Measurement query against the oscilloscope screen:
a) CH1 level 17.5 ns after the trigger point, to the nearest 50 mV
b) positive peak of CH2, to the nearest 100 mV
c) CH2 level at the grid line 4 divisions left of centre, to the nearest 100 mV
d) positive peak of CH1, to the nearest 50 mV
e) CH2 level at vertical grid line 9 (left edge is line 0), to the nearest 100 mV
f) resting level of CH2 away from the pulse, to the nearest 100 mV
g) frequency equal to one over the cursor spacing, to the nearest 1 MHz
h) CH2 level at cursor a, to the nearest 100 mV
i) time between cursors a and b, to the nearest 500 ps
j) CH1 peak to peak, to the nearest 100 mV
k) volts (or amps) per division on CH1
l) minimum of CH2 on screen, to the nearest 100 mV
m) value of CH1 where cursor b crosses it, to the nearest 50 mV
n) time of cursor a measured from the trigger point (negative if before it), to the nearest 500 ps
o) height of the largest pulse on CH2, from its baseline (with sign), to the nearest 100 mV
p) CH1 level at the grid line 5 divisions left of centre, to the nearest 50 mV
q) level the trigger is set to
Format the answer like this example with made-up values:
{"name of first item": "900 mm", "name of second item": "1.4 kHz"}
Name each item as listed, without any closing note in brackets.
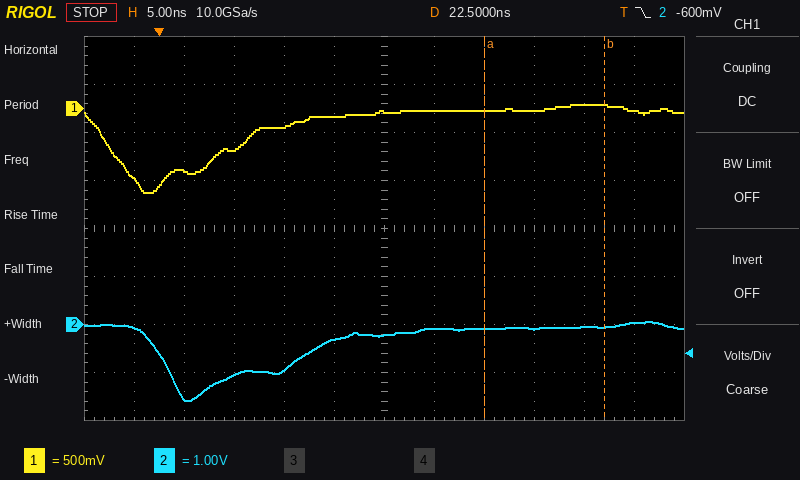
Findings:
{"CH1 level 17.5 ns after the trigger point, to the nearest 50 mV": "-100 mV", "positive peak of CH2, to the nearest 100 mV": "100 mV", "CH2 level at the grid line 4 divisions left of centre, to the nearest 100 mV": "-1.5 V", "positive peak of CH1, to the nearest 50 mV": "50 mV", "CH2 level at vertical grid line 9 (left edge is line 0), to the nearest 100 mV": "-100 mV", "resting level of CH2 away from the pulse, to the nearest 100 mV": "-100 mV", "frequency equal to one over the cursor spacing, to the nearest 1 MHz": "83 MHz", "CH2 level at cursor a, to the nearest 100 mV": "-100 mV", "time between cursors a and b, to the nearest 500 ps": "12.0 ns", "CH1 peak to peak, to the nearest 100 mV": "900 mV", "volts (or amps) per division on CH1": "500 mV", "minimum of CH2 on screen, to the nearest 100 mV": "-1.6 V", "value of CH1 where cursor b crosses it, to the nearest 50 mV": "50 mV", "time of cursor a measured from the trigger point (negative if before it), to the nearest 500 ps": "+32.5 ns", "height of the largest pulse on CH2, from its baseline (with sign), to the nearest 100 mV": "-1.5 V", "CH1 level at the grid line 5 divisions left of centre, to the nearest 50 mV": "-750 mV", "level the trigger is set to": "-600 mV"}
